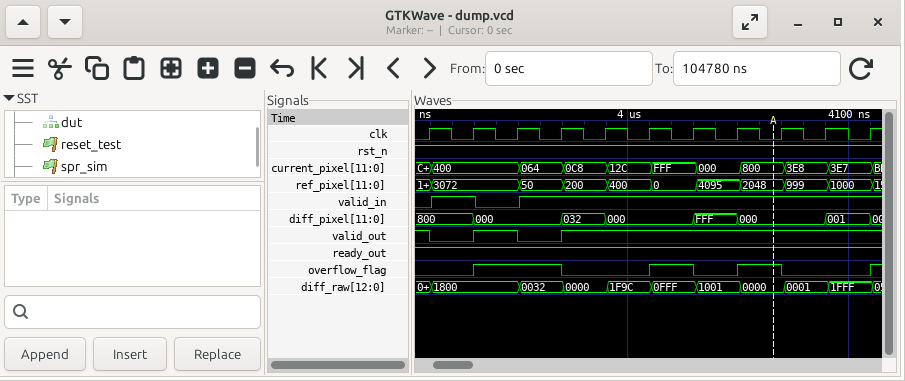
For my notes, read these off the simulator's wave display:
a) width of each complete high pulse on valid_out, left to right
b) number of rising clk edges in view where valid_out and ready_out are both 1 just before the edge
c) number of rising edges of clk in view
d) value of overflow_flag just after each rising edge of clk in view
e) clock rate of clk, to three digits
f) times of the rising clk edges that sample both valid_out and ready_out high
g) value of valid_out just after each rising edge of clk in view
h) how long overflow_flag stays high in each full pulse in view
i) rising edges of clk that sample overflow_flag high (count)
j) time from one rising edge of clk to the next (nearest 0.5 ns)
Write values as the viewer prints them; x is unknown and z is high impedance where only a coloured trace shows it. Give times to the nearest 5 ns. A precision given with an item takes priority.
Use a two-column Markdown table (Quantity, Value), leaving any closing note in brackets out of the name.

| Quantity | Value |
|---|---|
| width of each complete high pulse on valid_out, left to right | 20 ns |
| number of rising clk edges in view where valid_out and ready_out are both 1 just before the edge | 9 |
| number of rising edges of clk in view | 11 |
| value of overflow_flag just after each rising edge of clk in view | 0 1 1 0 0 1 0 1 0 0 1 |
| clock rate of clk, to three digits | 50.0 MHz |
| times of the rising clk edges that sample both valid_out and ready_out high | 3910 ns, 3950 ns, 3990 ns, 4010 ns, 4030 ns, 4050 ns, 4070 ns, 4090 ns, 4110 ns |
| value of valid_out just after each rising edge of clk in view | 0 1 0 1 1 1 1 1 1 1 1 |
| how long overflow_flag stays high in each full pulse in view | 40 ns, 20 ns, 20 ns |
| rising edges of clk that sample overflow_flag high | 4 |
| time from one rising edge of clk to the next | 20 ns |
